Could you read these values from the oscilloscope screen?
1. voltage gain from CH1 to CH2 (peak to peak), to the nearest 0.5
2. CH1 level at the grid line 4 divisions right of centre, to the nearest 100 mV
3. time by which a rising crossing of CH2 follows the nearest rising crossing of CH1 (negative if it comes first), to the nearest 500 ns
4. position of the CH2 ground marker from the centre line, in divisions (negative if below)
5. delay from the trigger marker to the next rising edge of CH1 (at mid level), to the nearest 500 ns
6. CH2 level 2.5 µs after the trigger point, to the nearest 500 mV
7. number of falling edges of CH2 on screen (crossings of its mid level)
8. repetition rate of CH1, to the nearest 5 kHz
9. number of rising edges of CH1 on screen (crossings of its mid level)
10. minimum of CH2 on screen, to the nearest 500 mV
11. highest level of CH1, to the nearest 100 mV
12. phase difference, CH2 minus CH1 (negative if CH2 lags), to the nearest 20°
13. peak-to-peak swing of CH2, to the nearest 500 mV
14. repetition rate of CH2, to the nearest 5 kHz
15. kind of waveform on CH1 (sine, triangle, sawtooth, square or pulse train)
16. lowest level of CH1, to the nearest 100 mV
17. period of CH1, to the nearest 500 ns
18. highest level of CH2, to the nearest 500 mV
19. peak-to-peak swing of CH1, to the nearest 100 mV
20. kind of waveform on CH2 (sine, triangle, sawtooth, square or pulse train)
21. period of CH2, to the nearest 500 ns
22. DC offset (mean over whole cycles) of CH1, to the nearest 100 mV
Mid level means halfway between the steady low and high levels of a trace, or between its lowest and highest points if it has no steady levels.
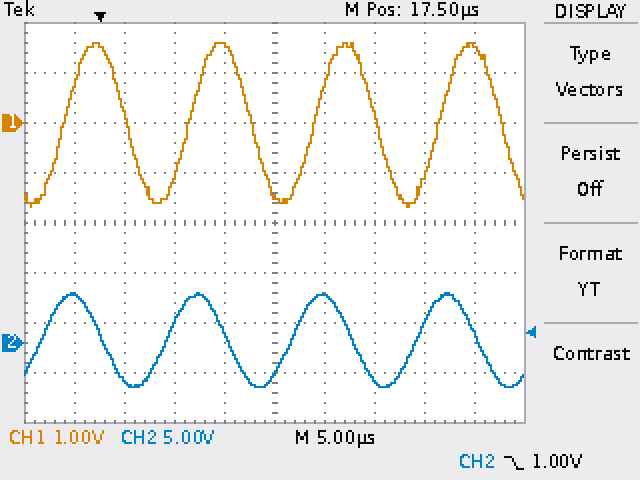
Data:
3.0
1.5 V
-2.0 µs
-2.4 div
9.0 µs
-4.0 V
4
80 kHz
4
-4.5 V
1.6 V
+60°
9.5 V
80 kHz
sine
-1.7 V
12.5 µs
5.0 V
3.3 V
sine
12.5 µs
0.0 V
